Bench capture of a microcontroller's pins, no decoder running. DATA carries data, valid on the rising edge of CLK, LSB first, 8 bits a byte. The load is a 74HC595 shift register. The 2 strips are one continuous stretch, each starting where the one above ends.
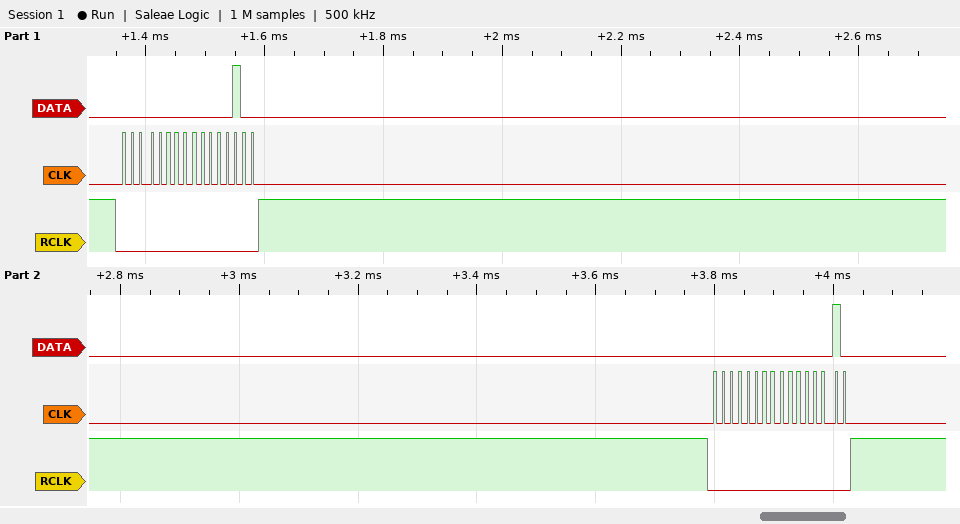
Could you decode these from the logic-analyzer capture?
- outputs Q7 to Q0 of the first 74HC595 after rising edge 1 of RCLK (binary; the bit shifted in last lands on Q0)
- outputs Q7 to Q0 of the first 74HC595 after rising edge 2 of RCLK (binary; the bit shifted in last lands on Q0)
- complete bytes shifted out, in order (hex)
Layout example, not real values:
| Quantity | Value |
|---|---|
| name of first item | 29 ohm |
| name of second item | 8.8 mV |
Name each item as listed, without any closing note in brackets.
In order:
| Quantity | Value |
|---|---|
| outputs Q7 to Q0 of the first 74HC595 after rising edge 1 of RCLK | 00000100 |
| outputs Q7 to Q0 of the first 74HC595 after rising edge 2 of RCLK | 00000010 |
| complete bytes shifted out, in order | 00 20 00 40 |
